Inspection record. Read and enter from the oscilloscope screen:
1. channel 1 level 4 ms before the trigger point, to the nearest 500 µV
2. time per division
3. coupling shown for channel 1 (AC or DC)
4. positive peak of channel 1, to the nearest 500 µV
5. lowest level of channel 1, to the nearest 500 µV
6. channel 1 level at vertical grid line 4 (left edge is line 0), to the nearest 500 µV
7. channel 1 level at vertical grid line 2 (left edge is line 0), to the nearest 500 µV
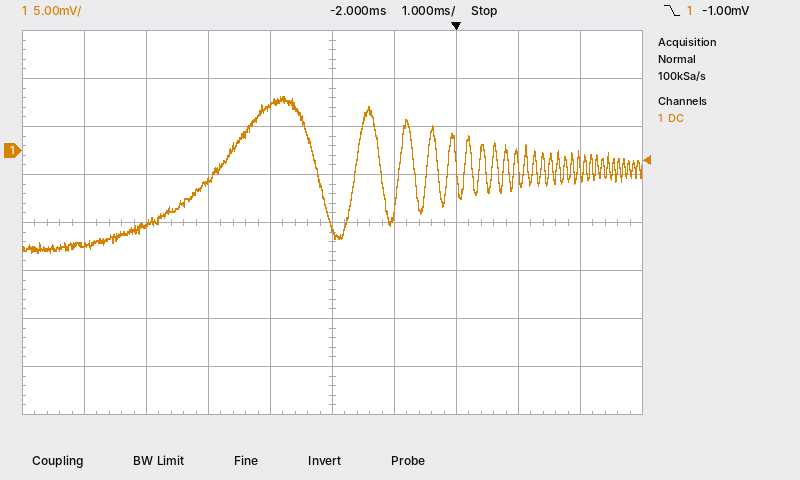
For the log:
-3.0 mV
1 ms
DC
5.5 mV
-10.5 mV
4.5 mV
-7.5 mV
